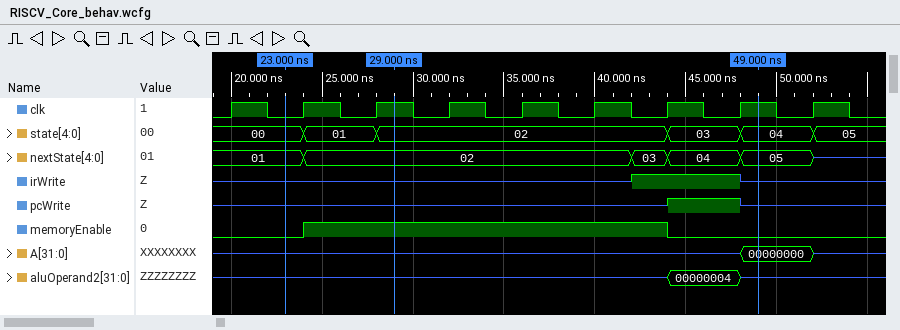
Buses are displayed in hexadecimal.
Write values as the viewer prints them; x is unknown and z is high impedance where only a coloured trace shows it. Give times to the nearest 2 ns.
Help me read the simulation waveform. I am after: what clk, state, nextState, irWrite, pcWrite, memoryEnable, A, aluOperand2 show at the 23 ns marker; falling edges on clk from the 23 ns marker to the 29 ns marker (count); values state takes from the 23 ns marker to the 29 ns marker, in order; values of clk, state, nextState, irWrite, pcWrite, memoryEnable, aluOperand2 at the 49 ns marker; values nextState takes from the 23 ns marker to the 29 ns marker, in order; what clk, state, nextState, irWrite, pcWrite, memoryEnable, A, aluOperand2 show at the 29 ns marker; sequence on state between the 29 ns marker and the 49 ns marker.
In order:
clk=0, state=00, nextState=01, irWrite=z, pcWrite=z, memoryEnable=0, A=z, aluOperand2=z
1
00, 01, 02
clk=1, state=04, nextState=05, irWrite=z, pcWrite=z, memoryEnable=0, aluOperand2=z
01, 02
clk=1, state=02, nextState=02, irWrite=z, pcWrite=z, memoryEnable=1, A=z, aluOperand2=z
02, 03, 04
